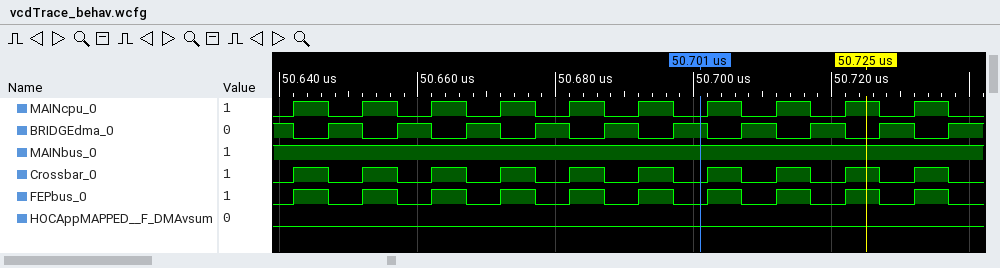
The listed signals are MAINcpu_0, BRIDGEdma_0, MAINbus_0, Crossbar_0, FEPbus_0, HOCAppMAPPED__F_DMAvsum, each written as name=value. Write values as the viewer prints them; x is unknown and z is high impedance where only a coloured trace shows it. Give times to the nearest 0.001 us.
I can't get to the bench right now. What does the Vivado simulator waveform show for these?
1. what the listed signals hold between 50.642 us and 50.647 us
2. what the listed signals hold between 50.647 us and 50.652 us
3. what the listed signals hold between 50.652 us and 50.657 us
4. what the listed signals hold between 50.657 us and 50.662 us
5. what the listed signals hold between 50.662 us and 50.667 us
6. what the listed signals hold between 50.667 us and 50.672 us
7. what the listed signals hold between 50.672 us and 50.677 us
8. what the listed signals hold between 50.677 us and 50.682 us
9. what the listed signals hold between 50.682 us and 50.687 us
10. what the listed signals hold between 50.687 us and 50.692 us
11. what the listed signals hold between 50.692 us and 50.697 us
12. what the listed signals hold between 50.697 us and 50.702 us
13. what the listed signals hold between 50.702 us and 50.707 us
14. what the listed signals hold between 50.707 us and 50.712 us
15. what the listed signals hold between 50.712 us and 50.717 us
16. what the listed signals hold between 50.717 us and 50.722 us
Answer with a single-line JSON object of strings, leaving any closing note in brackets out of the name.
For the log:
{"what the listed signals hold between 50.642 us and 50.647 us": "MAINcpu_0=1, BRIDGEdma_0=0, MAINbus_0=1, Crossbar_0=1, FEPbus_0=1, HOCAppMAPPED__F_DMAvsum=0", "what the listed signals hold between 50.647 us and 50.652 us": "MAINcpu_0=0, BRIDGEdma_0=1, MAINbus_0=1, Crossbar_0=0, FEPbus_0=0, HOCAppMAPPED__F_DMAvsum=0", "what the listed signals hold between 50.652 us and 50.657 us": "MAINcpu_0=1, BRIDGEdma_0=0, MAINbus_0=1, Crossbar_0=1, FEPbus_0=1, HOCAppMAPPED__F_DMAvsum=0", "what the listed signals hold between 50.657 us and 50.662 us": "MAINcpu_0=0, BRIDGEdma_0=1, MAINbus_0=1, Crossbar_0=0, FEPbus_0=0, HOCAppMAPPED__F_DMAvsum=0", "what the listed signals hold between 50.662 us and 50.667 us": "MAINcpu_0=1, BRIDGEdma_0=0, MAINbus_0=1, Crossbar_0=1, FEPbus_0=1, HOCAppMAPPED__F_DMAvsum=0", "what the listed signals hold between 50.667 us and 50.672 us": "MAINcpu_0=0, BRIDGEdma_0=1, MAINbus_0=1, Crossbar_0=0, FEPbus_0=0, HOCAppMAPPED__F_DMAvsum=0", "what the listed signals hold between 50.672 us and 50.677 us": "MAINcpu_0=1, BRIDGEdma_0=0, MAINbus_0=1, Crossbar_0=1, FEPbus_0=1, HOCAppMAPPED__F_DMAvsum=0", "what the listed signals hold between 50.677 us and 50.682 us": "MAINcpu_0=0, BRIDGEdma_0=1, MAINbus_0=1, Crossbar_0=0, FEPbus_0=0, HOCAppMAPPED__F_DMAvsum=0", "what the listed signals hold between 50.682 us and 50.687 us": "MAINcpu_0=1, BRIDGEdma_0=0, MAINbus_0=1, Crossbar_0=1, FEPbus_0=1, HOCAppMAPPED__F_DMAvsum=0", "what the listed signals hold between 50.687 us and 50.692 us": "MAINcpu_0=0, BRIDGEdma_0=1, MAINbus_0=1, Crossbar_0=0, FEPbus_0=0, HOCAppMAPPED__F_DMAvsum=0", "what the listed signals hold between 50.692 us and 50.697 us": "MAINcpu_0=1, BRIDGEdma_0=0, MAINbus_0=1, Crossbar_0=1, FEPbus_0=1, HOCAppMAPPED__F_DMAvsum=0", "what the listed signals hold between 50.697 us and 50.702 us": "MAINcpu_0=0, BRIDGEdma_0=1, MAINbus_0=1, Crossbar_0=0, FEPbus_0=0, HOCAppMAPPED__F_DMAvsum=0", "what the listed signals hold between 50.702 us and 50.707 us": "MAINcpu_0=1, BRIDGEdma_0=0, MAINbus_0=1, Crossbar_0=1, FEPbus_0=1, HOCAppMAPPED__F_DMAvsum=0", "what the listed signals hold between 50.707 us and 50.712 us": "MAINcpu_0=0, BRIDGEdma_0=1, MAINbus_0=1, Crossbar_0=0, FEPbus_0=0, HOCAppMAPPED__F_DMAvsum=0", "what the listed signals hold between 50.712 us and 50.717 us": "MAINcpu_0=1, BRIDGEdma_0=0, MAINbus_0=1, Crossbar_0=1, FEPbus_0=1, HOCAppMAPPED__F_DMAvsum=0", "what the listed signals hold between 50.717 us and 50.722 us": "MAINcpu_0=0, BRIDGEdma_0=1, MAINbus_0=1, Crossbar_0=0, FEPbus_0=0, HOCAppMAPPED__F_DMAvsum=0"}
